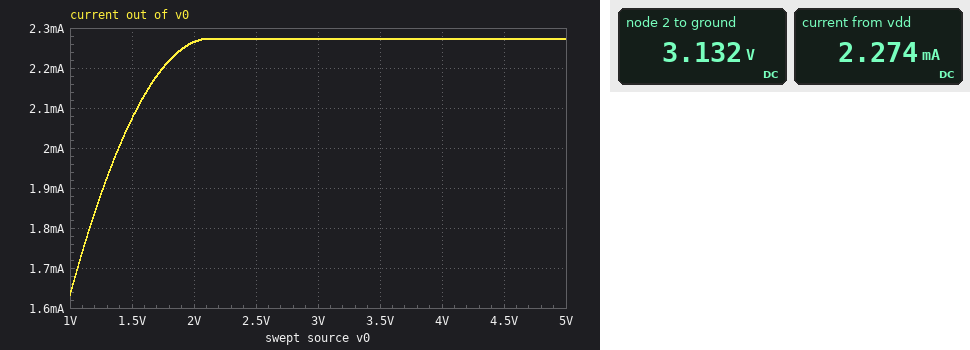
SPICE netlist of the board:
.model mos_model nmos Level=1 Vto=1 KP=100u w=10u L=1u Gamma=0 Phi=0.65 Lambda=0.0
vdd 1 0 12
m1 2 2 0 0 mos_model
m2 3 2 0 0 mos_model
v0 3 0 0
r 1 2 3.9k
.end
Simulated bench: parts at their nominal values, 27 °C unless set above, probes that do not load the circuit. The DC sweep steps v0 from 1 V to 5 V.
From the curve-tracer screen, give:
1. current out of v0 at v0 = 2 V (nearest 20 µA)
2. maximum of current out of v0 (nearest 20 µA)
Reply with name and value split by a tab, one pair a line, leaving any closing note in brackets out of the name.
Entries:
current out of v0 at v0 = 2 V	2.26 mA
maximum of current out of v0	2.28 mA
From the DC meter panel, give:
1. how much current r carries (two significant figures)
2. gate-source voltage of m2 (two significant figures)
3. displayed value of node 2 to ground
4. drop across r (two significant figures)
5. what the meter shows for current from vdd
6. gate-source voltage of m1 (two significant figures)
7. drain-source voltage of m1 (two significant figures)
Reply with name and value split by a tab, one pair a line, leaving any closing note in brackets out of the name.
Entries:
how much current r carries	2.3 mA
gate-source voltage of m2	3.1 V
displayed value of node 2 to ground	3.132 V
drop across r	8.9 V
what the meter shows for current from vdd	2.274 mA
gate-source voltage of m1	3.1 V
drain-source voltage of m1	3.1 V
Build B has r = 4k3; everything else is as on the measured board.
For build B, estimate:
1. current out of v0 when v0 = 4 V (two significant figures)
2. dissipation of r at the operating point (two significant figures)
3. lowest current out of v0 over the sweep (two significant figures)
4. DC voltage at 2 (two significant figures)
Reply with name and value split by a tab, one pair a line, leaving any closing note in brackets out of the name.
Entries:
current out of v0 when v0 = 4 V	2.1 mA
dissipation of r at the operating point	19 mW
lowest current out of v0 over the sweep	1.5 mA
DC voltage at 2	3.0 V
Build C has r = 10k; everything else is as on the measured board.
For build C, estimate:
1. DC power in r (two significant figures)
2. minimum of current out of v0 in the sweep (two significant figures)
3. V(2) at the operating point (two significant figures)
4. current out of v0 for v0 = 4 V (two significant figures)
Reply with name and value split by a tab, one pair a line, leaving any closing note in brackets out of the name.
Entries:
DC power in r	9.2 mW
minimum of current out of v0 in the sweep	890 µA
V(2) at the operating point	2.4 V
current out of v0 for v0 = 4 V	960 µA
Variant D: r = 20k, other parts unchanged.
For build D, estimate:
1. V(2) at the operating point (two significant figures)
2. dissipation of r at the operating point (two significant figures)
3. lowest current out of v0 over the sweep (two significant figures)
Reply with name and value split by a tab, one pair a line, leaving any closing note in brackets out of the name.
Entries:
V(2) at the operating point	2.0 V
dissipation of r at the operating point	5.0 mW
lowest current out of v0 over the sweep	500 µA
